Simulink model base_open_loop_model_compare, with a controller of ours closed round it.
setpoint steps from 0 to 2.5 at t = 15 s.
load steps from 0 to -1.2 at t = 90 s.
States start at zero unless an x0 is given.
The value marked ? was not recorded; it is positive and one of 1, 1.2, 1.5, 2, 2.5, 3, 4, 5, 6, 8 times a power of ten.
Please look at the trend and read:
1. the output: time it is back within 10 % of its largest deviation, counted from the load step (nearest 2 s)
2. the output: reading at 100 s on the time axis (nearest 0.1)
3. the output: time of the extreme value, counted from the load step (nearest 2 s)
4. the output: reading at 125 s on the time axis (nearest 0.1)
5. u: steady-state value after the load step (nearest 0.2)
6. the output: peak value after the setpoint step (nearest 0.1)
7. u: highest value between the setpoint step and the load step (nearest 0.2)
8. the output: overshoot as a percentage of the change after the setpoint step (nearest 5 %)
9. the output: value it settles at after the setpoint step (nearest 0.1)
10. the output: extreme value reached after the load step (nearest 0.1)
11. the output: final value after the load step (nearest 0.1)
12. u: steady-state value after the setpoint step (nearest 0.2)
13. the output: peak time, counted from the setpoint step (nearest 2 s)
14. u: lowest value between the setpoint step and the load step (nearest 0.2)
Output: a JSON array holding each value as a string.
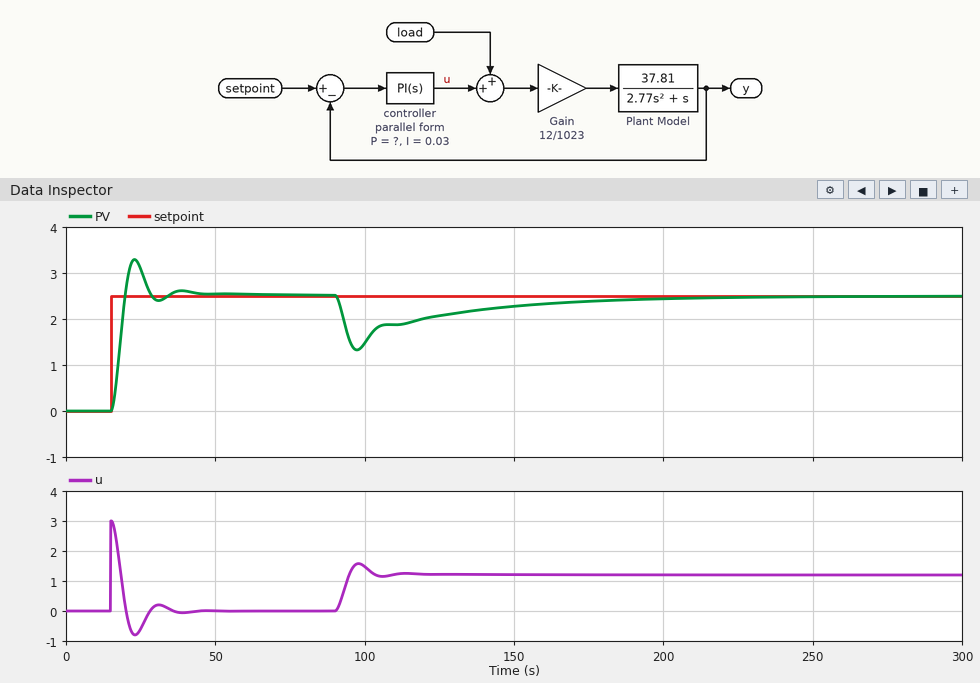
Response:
["84 s", "1.5", "8 s", "2.1", "1.2", "3.3", "3.0", "30 %", "2.5", "1.3", "2.5", "0.0", "8 s", "-0.8"]
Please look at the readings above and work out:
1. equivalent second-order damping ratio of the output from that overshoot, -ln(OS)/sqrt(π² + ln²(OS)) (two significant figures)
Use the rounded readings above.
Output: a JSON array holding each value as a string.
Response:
["0.36"]
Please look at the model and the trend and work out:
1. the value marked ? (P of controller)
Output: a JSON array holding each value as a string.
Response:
["1.2"]
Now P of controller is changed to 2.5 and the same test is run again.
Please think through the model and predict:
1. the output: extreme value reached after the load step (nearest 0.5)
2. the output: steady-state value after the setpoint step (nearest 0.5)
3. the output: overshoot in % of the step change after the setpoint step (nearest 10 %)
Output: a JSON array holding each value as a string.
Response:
["2.0", "2.5", "40 %"]
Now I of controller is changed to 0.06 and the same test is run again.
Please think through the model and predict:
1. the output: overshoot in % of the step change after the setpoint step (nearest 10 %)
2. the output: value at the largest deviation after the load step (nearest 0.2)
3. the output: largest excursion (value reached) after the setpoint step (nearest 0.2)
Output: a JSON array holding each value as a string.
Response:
["40 %", "1.4", "3.4"]
